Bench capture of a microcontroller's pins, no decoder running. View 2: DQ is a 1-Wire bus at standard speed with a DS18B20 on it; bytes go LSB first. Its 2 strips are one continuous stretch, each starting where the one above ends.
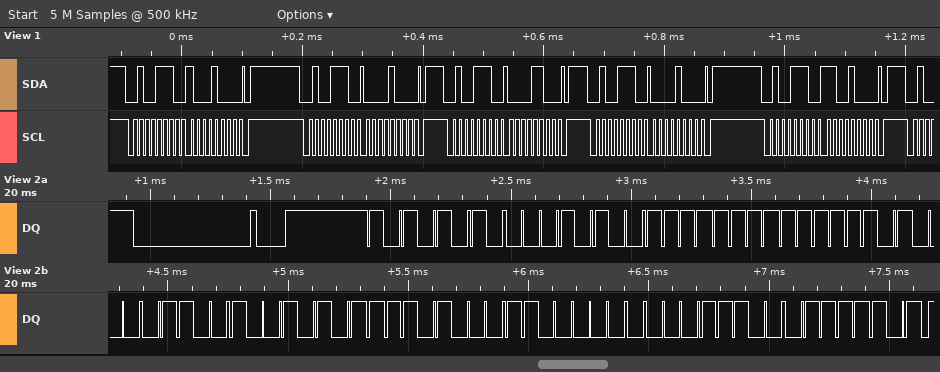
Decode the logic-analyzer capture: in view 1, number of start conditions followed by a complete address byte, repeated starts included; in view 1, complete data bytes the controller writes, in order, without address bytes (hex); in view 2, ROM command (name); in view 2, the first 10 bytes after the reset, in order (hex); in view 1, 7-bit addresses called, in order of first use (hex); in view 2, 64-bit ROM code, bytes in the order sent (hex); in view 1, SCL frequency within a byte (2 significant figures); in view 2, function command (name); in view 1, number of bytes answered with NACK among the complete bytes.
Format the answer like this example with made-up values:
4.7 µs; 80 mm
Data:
5; 88 08 0C 08 C8; Match ROM; 55 28 FF BF 30 A9 17 03 38 BE; 0x27; 28 FF BF 30 A9 17 03 38; 100 kHz; Read Scratchpad; 0
